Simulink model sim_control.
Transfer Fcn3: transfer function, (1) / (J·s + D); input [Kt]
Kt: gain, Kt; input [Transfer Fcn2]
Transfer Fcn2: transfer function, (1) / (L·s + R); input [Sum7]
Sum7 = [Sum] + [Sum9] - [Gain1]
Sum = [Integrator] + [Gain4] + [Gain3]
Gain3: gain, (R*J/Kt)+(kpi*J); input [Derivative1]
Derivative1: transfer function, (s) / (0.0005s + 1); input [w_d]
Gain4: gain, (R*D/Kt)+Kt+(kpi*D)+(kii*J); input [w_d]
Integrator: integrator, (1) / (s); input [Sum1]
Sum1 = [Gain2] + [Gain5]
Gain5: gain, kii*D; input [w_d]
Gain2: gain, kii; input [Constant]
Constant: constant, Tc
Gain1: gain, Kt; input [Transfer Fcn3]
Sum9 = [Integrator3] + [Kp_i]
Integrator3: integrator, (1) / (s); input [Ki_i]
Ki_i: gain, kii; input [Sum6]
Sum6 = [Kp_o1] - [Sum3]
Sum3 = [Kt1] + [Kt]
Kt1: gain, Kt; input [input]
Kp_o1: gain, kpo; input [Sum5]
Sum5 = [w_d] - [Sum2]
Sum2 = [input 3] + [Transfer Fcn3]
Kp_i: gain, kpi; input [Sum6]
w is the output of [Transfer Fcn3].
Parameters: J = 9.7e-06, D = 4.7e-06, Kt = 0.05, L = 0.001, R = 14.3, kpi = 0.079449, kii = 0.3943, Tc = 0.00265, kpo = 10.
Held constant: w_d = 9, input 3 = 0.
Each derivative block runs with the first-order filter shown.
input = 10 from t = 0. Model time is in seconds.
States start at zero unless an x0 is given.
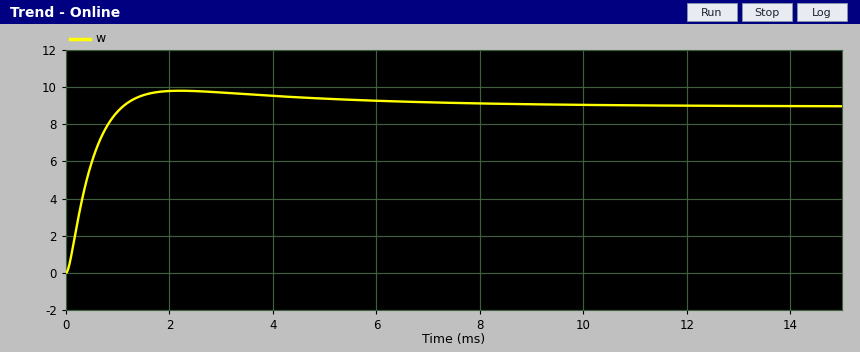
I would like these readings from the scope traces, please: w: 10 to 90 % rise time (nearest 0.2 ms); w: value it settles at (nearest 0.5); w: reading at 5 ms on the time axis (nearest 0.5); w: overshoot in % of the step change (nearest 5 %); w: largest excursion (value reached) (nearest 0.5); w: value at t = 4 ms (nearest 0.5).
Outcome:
0.8 ms
9.0
9.5
10 %
10.0
9.5
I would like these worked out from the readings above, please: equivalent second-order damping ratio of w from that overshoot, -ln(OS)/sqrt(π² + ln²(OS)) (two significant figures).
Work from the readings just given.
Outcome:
0.59
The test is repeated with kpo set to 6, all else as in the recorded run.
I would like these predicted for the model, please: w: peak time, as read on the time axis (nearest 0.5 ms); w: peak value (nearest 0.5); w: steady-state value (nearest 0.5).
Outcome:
2.5 ms
9.5
9.0
